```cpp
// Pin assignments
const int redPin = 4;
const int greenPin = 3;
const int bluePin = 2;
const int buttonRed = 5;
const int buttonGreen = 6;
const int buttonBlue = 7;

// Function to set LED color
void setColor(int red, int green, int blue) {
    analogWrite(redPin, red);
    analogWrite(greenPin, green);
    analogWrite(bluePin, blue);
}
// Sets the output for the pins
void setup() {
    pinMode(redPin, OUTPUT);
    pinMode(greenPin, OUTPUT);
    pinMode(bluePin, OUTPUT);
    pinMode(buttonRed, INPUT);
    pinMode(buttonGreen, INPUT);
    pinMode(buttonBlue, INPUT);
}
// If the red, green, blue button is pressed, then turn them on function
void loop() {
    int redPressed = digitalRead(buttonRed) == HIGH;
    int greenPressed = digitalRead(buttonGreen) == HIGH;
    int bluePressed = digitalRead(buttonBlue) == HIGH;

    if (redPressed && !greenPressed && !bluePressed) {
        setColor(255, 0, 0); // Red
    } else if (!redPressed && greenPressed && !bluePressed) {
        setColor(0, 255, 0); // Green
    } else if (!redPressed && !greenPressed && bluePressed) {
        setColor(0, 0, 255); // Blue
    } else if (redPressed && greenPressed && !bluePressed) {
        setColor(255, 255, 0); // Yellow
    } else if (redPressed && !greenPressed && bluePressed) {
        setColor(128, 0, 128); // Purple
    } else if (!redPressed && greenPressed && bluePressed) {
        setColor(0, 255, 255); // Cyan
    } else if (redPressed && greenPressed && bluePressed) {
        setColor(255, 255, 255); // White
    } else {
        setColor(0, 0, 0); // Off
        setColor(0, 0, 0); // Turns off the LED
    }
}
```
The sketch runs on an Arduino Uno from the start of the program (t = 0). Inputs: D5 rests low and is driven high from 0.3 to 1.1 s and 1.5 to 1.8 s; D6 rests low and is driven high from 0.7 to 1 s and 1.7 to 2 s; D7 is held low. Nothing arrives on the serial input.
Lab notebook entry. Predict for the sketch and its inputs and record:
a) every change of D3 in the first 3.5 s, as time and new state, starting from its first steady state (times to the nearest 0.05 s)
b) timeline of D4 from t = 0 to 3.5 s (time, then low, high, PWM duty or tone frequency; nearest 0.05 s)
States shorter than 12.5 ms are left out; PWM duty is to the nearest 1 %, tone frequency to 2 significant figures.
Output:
0 s low; 0.7 s high; 1 s low; 1.7 s high; 2 s low
0 s low; 0.3 s high; 1.1 s low; 1.5 s high; 1.8 s low
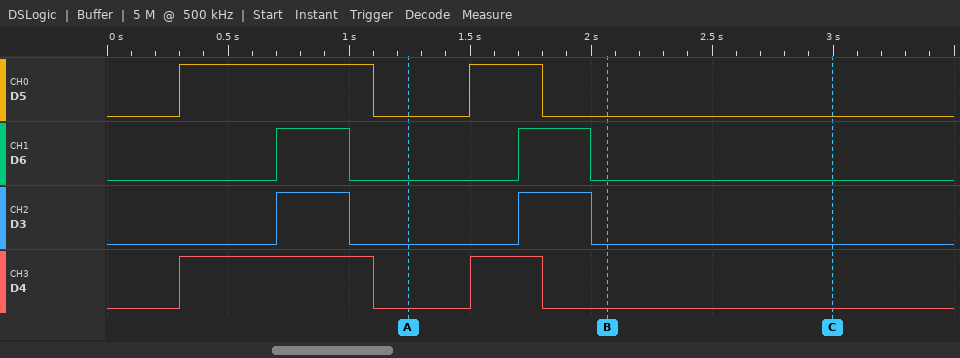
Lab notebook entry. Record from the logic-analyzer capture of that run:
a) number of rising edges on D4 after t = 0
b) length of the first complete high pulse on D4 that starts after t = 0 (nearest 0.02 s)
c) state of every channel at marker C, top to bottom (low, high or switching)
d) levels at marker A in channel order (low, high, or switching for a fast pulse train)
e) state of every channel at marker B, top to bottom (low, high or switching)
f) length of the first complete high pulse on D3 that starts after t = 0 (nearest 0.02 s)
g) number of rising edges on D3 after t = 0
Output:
2
0.80 s
D5 low, D6 low, D3 low, D4 low
D5 low, D6 low, D3 low, D4 low
D5 low, D6 low, D3 low, D4 low
0.30 s
2
